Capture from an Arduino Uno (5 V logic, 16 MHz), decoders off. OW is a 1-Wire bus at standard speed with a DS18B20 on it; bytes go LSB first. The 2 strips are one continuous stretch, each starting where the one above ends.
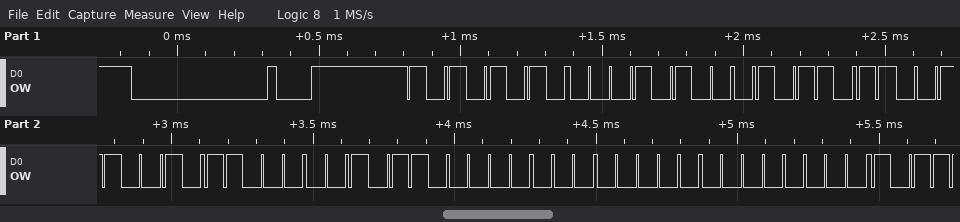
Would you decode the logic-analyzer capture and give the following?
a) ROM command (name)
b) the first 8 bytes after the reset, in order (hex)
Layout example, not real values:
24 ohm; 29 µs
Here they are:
Match ROM; 55 28 DA 4C 83 06 00 00
